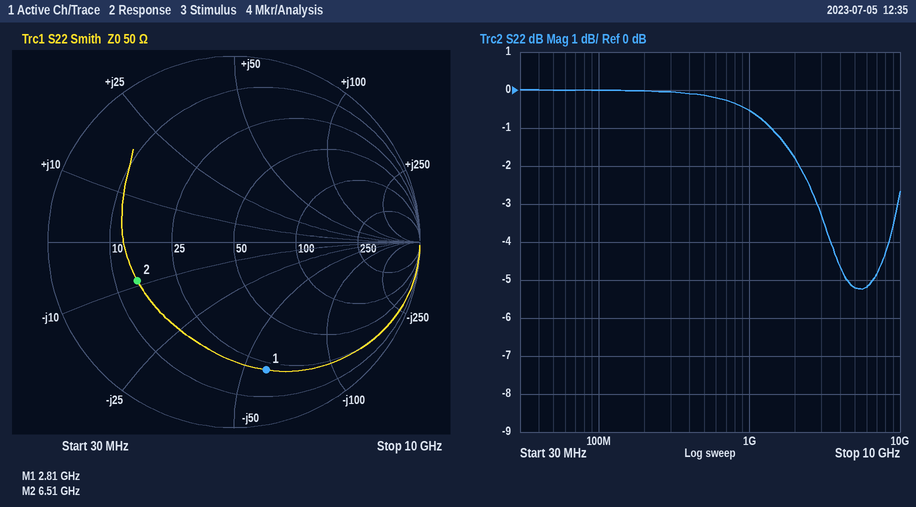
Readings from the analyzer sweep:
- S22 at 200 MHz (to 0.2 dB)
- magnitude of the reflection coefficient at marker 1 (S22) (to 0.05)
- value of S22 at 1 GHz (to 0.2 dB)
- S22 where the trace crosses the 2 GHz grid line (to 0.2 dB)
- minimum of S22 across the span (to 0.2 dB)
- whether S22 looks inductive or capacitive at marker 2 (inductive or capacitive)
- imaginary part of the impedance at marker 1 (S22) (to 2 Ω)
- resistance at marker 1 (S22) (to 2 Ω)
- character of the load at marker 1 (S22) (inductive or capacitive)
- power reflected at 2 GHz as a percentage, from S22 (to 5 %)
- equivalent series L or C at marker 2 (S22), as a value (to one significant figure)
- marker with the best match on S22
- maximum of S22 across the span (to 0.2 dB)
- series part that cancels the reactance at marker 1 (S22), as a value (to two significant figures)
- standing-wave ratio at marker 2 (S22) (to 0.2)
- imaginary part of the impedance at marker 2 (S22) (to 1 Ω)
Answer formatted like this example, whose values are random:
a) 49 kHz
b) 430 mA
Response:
a) 0.0 dB
b) 0.70
c) -0.6 dB
d) -1.8 dB
e) -5.2 dB
f) capacitive
g) -60 Ω
h) 22 Ω
i) capacitive
j) 65 %
k) 3 pF
l) marker 2
m) 0.0 dB
n) 3.4 nH
o) 3.6
p) -9 Ω
